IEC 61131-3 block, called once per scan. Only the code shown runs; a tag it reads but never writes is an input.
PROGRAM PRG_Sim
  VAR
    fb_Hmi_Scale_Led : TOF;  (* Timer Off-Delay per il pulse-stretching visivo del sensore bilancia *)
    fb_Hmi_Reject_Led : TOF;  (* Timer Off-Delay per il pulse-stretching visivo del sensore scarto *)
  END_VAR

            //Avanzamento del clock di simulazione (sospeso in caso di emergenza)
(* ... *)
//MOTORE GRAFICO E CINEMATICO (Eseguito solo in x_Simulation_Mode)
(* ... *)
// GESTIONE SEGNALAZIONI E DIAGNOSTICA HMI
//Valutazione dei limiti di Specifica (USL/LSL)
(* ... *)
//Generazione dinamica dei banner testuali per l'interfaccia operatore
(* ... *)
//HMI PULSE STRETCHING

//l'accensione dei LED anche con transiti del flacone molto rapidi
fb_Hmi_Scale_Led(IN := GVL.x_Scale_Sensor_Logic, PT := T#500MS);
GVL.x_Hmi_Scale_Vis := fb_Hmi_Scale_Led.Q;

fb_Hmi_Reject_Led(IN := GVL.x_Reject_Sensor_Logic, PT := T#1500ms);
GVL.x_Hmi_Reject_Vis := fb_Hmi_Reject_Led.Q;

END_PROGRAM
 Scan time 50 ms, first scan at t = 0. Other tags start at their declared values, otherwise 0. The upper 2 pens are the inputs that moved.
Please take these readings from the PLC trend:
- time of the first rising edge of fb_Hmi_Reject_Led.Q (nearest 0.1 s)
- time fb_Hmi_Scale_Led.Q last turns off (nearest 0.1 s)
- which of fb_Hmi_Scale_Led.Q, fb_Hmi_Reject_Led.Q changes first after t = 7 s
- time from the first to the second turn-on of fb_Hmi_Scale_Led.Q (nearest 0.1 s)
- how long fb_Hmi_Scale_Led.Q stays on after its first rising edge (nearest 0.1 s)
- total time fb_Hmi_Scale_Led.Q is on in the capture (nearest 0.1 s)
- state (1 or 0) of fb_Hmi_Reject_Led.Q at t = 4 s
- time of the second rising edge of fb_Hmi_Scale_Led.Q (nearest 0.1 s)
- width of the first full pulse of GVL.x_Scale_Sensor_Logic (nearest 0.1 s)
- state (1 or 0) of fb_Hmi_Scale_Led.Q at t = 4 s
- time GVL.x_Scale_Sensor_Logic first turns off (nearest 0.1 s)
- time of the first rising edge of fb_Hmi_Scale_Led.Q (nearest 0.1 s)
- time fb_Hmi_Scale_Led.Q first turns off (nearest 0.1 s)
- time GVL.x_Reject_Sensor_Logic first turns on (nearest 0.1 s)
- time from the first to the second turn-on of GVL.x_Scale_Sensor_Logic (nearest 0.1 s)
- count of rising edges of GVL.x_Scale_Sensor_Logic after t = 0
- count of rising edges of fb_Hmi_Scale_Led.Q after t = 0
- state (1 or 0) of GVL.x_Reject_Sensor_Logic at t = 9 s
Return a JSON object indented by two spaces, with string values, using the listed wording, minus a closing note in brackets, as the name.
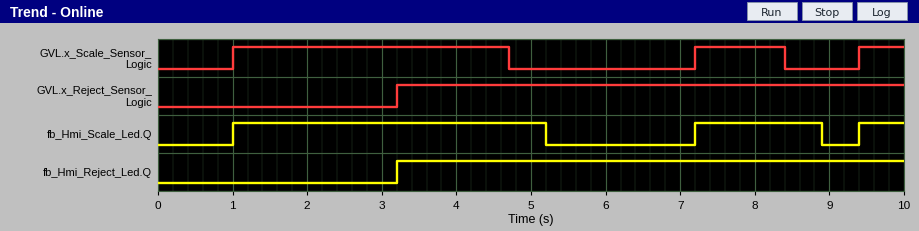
{
  "time of the first rising edge of fb_Hmi_Reject_Led.Q": "3.2 s",
  "time fb_Hmi_Scale_Led.Q last turns off": "8.9 s",
  "which of fb_Hmi_Scale_Led.Q, fb_Hmi_Reject_Led.Q changes first after t = 7 s": "fb_Hmi_Scale_Led.Q",
  "time from the first to the second turn-on of fb_Hmi_Scale_Led.Q": "6.2 s",
  "how long fb_Hmi_Scale_Led.Q stays on after its first rising edge": "4.2 s",
  "total time fb_Hmi_Scale_Led.Q is on in the capture": "6.5 s",
  "state (1 or 0) of fb_Hmi_Reject_Led.Q at t = 4 s": "1",
  "time of the second rising edge of fb_Hmi_Scale_Led.Q": "7.2 s",
  "width of the first full pulse of GVL.x_Scale_Sensor_Logic": "3.7 s",
  "state (1 or 0) of fb_Hmi_Scale_Led.Q at t = 4 s": "1",
  "time GVL.x_Scale_Sensor_Logic first turns off": "4.7 s",
  "time of the first rising edge of fb_Hmi_Scale_Led.Q": "1.0 s",
  "time fb_Hmi_Scale_Led.Q first turns off": "5.2 s",
  "time GVL.x_Reject_Sensor_Logic first turns on": "3.2 s",
  "time from the first to the second turn-on of GVL.x_Scale_Sensor_Logic": "6.2 s",
  "count of rising edges of GVL.x_Scale_Sensor_Logic after t = 0": "3",
  "count of rising edges of fb_Hmi_Scale_Led.Q after t = 0": "3",
  "state (1 or 0) of GVL.x_Reject_Sensor_Logic at t = 9 s": "1"
}
